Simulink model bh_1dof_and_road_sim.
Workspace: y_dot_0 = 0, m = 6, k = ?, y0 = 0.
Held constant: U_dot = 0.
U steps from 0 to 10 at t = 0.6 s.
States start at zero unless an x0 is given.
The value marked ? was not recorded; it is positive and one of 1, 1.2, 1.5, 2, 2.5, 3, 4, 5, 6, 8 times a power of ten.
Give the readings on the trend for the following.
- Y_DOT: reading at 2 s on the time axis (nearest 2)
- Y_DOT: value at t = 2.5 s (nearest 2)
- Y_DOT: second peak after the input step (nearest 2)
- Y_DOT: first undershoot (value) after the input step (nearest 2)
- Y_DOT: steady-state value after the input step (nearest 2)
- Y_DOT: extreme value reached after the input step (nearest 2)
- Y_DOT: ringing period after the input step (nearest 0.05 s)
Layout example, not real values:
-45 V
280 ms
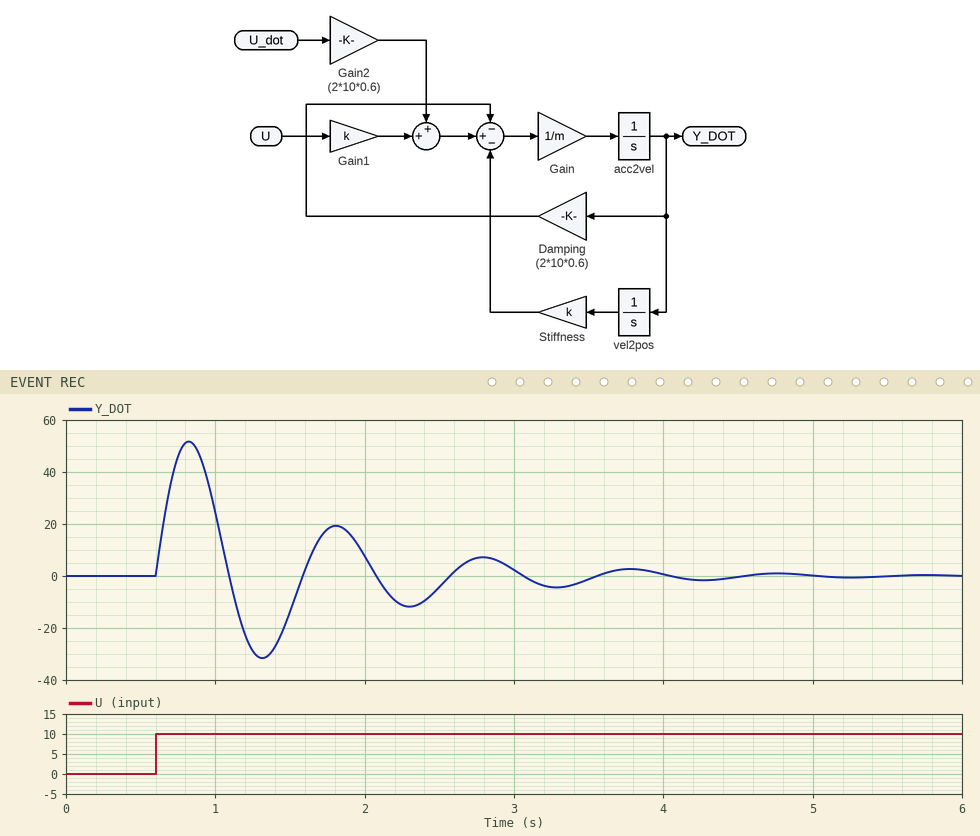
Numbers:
8
-4
20
-32
0
52
1.00 s
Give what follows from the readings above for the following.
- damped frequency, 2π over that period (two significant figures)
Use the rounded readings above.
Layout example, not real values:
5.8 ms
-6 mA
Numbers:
6.3 rad/s
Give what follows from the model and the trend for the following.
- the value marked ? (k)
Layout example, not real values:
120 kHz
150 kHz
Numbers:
250
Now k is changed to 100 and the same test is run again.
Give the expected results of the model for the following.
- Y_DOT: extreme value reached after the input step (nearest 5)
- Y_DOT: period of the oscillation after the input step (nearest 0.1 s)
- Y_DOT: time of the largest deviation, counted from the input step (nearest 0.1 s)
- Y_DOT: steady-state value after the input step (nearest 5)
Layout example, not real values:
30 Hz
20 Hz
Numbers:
30
1.6 s
0.3 s
0
